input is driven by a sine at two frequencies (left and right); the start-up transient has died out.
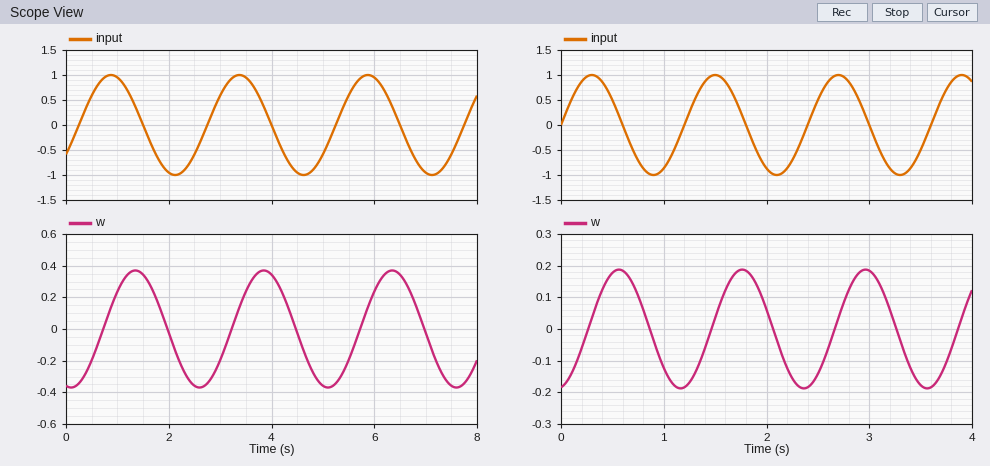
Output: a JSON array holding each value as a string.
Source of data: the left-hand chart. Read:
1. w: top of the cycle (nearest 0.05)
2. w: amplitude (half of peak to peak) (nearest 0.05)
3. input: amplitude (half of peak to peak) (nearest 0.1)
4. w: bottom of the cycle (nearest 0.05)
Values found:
["0.35", "0.35", "1.0", "-0.35"]
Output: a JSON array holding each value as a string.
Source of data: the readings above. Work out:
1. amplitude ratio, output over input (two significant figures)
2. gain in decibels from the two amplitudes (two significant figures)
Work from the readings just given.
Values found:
["0.35", "-9.1 dB"]
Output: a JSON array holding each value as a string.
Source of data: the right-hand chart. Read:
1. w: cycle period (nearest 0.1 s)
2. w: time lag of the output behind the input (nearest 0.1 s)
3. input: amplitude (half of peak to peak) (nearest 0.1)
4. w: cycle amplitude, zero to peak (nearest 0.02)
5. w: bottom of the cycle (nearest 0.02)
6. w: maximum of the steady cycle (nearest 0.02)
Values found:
["1.2 s", "0.3 s", "1.0", "0.18", "-0.18", "0.18"]
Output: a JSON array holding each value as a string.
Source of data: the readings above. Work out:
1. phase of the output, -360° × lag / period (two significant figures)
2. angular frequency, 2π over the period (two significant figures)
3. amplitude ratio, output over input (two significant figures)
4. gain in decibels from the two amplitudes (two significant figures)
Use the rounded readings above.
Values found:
["-90°", "5.2 rad/s", "0.18", "-15 dB"]
